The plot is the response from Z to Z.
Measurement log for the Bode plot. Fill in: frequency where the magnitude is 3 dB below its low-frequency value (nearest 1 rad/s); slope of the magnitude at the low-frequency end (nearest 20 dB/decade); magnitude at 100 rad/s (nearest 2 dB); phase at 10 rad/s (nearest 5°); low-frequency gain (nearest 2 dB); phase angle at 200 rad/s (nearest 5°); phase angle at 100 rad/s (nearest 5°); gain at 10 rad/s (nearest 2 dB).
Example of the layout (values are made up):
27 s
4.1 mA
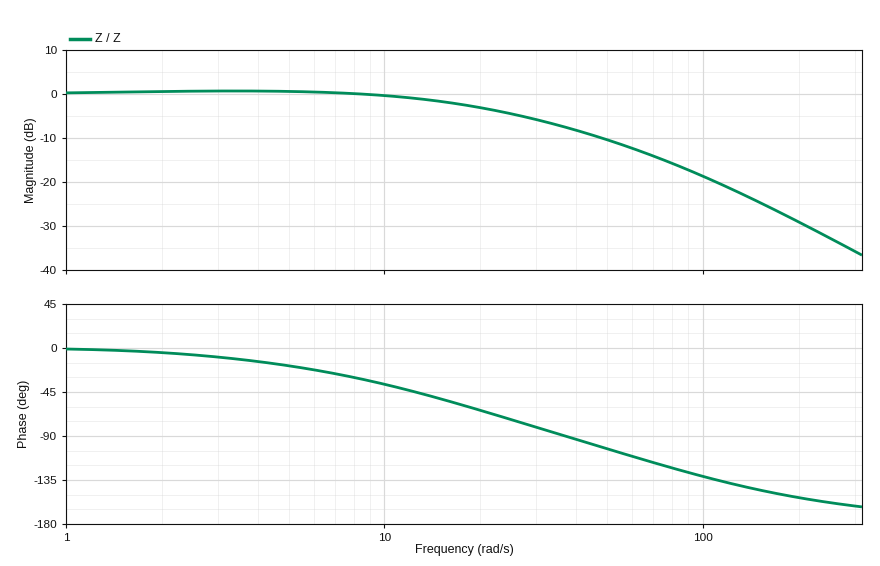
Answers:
18 rad/s
0 dB/decade
-18 dB
-35°
0 dB
-155°
-130°
0 dB
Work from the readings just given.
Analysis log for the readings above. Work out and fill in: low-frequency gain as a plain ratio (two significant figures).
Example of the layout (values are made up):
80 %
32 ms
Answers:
1.0
